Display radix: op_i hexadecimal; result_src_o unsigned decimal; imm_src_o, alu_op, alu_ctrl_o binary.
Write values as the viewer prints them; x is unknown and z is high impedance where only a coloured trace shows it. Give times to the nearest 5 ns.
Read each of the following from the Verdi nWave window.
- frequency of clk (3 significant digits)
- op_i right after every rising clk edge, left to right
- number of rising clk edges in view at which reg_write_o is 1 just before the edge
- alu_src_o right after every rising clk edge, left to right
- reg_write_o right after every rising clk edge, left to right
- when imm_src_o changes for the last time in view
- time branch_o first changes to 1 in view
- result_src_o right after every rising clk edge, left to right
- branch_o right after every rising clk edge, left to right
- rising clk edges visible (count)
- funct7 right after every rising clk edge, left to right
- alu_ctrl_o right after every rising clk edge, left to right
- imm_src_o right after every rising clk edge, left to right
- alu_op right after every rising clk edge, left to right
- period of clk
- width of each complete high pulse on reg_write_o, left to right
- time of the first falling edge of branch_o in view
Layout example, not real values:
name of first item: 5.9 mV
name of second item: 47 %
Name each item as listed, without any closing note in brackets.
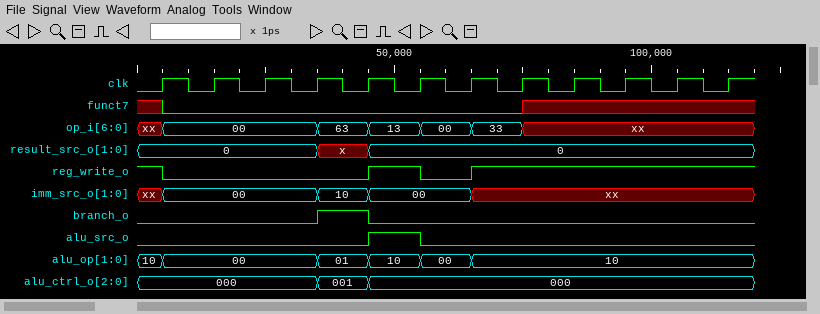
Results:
frequency of clk: 100 MHz
op_i right after every rising clk edge, left to right: 00, 00, 00, 63, 13, 00, 33, xx, xx, xx, xx, xx
number of rising clk edges in view at which reg_write_o is 1 just before the edge: 7
alu_src_o right after every rising clk edge, left to right: 0 0 0 0 1 0 0 0 0 0 0 0
reg_write_o right after every rising clk edge, left to right: 0 0 0 0 1 0 1 1 1 1 1 1
when imm_src_o changes for the last time in view: 65 ns
time branch_o first changes to 1 in view: 35 ns
result_src_o right after every rising clk edge, left to right: 0, 0, 0, x, 0, 0, 0, 0, 0, 0, 0, 0
branch_o right after every rising clk edge, left to right: 0 0 0 1 0 0 0 0 0 0 0 0
rising clk edges visible: 12
funct7 right after every rising clk edge, left to right: 0 0 0 0 0 0 0 x x x x x
alu_ctrl_o right after every rising clk edge, left to right: 000, 000, 000, 001, 000, 000, 000, 000, 000, 000, 000, 000
imm_src_o right after every rising clk edge, left to right: 00, 00, 00, 10, 00, 00, xx, xx, xx, xx, xx, xx
alu_op right after every rising clk edge, left to right: 00, 00, 00, 01, 10, 00, 10, 10, 10, 10, 10, 10
period of clk: 10 ns
width of each complete high pulse on reg_write_o, left to right: 10 ns
time of the first falling edge of branch_o in view: 45 ns
